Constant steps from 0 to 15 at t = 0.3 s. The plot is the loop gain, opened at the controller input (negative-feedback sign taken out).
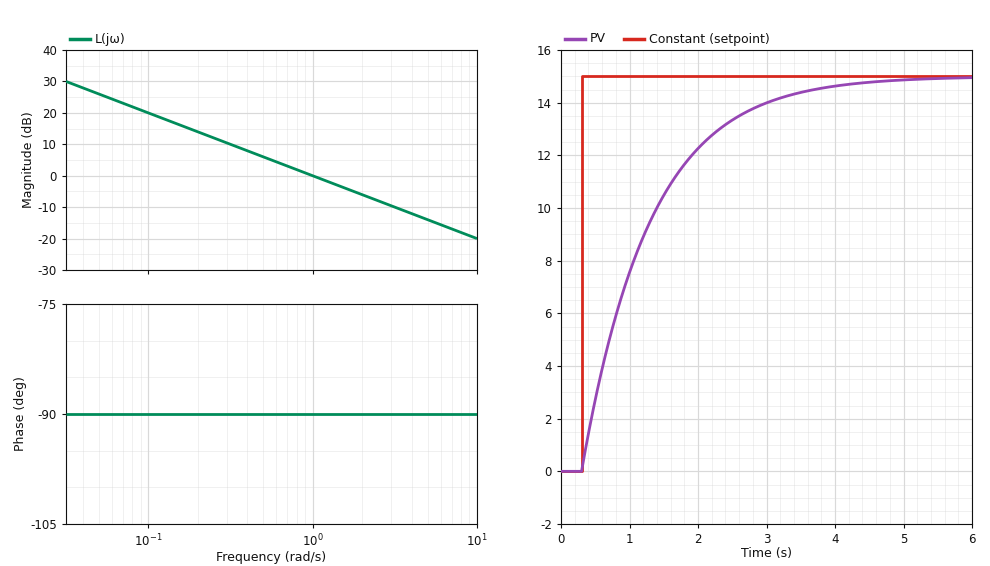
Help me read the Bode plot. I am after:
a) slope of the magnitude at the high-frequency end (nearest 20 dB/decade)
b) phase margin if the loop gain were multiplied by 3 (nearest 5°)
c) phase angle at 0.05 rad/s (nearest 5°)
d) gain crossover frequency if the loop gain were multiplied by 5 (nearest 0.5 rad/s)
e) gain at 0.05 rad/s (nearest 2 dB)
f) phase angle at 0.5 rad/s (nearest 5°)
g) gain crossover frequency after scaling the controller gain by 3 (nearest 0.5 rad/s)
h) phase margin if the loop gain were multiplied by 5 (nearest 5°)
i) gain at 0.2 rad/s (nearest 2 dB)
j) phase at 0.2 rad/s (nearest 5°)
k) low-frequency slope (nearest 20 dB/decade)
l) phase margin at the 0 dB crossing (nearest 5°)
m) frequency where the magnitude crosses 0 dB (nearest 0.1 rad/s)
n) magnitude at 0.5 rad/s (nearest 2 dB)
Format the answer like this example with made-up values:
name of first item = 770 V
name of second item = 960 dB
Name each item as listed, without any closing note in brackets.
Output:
slope of the magnitude at the high-frequency end = -20 dB/decade
phase margin if the loop gain were multiplied by 3 = 90°
phase angle at 0.05 rad/s = -90°
gain crossover frequency if the loop gain were multiplied by 5 = 5.0 rad/s
gain at 0.05 rad/s = 26 dB
phase angle at 0.5 rad/s = -90°
gain crossover frequency after scaling the controller gain by 3 = 3.0 rad/s
phase margin if the loop gain were multiplied by 5 = 90°
gain at 0.2 rad/s = 14 dB
phase at 0.2 rad/s = -90°
low-frequency slope = -20 dB/decade
phase margin at the 0 dB crossing = 90°
frequency where the magnitude crosses 0 dB = 1.0 rad/s
magnitude at 0.5 rad/s = 6 dB
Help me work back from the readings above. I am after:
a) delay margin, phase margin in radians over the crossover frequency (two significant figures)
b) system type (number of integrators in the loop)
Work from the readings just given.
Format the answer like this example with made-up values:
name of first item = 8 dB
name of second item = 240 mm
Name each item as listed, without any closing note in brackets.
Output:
delay margin, phase margin in radians over the crossover frequency = 1.6 s
system type = 1
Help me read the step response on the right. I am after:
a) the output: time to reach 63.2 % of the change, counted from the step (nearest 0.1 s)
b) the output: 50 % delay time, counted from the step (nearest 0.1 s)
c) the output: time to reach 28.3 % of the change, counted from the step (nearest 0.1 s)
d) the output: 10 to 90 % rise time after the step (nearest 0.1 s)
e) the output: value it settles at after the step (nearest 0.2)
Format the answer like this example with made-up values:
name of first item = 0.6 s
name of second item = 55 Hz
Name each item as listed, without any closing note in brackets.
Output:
the output: time to reach 63.2 % of the change, counted from the step = 1.0 s
the output: 50 % delay time, counted from the step = 0.7 s
the output: time to reach 28.3 % of the change, counted from the step = 0.3 s
the output: 10 to 90 % rise time after the step = 2.2 s
the output: value it settles at after the step = 15.0
